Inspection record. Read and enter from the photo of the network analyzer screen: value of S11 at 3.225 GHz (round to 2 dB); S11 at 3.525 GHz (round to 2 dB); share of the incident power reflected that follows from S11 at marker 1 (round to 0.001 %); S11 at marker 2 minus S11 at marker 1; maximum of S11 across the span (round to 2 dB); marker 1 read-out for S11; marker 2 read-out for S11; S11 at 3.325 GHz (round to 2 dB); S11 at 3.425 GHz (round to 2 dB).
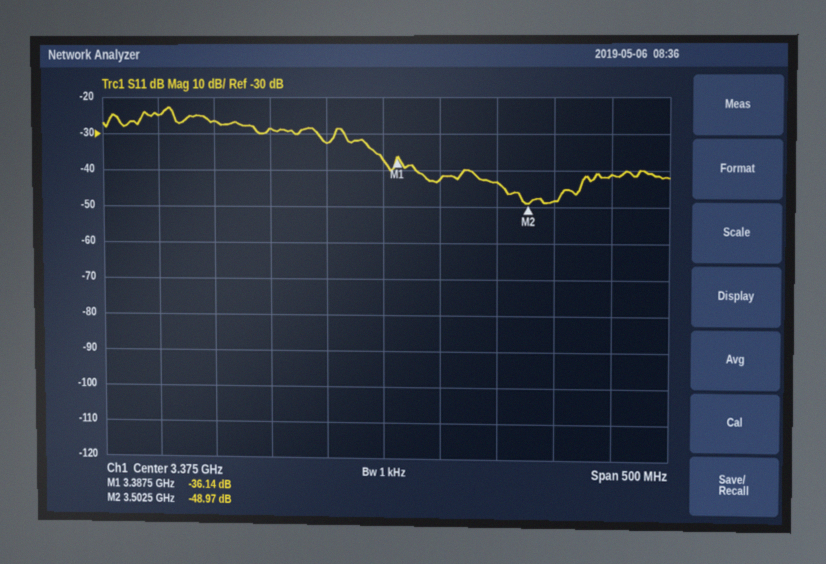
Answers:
-26 dB
-48 dB
0.024 %
-12.83 dB
-22 dB
-36.14 dB
-48.97 dB
-32 dB
-42 dB
